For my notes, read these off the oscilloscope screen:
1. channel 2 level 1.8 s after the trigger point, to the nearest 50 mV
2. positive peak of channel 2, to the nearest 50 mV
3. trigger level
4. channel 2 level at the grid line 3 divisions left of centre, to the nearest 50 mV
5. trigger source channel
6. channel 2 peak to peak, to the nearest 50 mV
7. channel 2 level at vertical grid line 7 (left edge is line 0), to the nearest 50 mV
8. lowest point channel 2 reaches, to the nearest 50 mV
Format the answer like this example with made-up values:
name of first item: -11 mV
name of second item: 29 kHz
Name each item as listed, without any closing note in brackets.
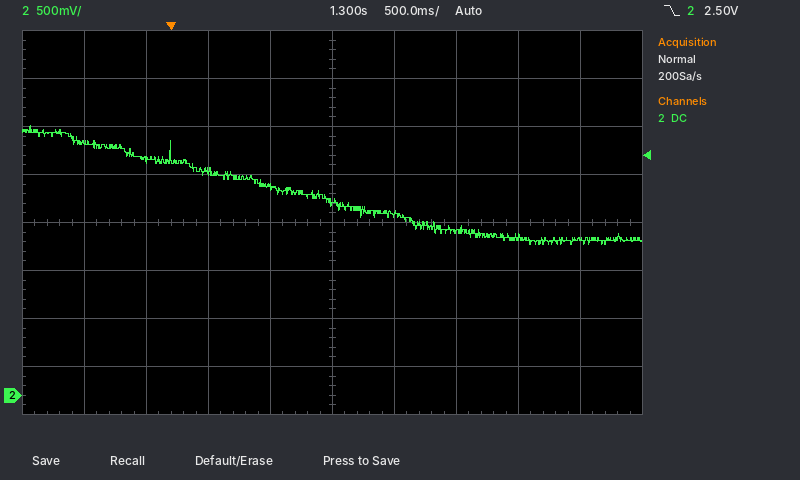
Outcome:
channel 2 level 1.8 s after the trigger point, to the nearest 50 mV: 1.90 V
positive peak of channel 2, to the nearest 50 mV: 2.80 V
trigger level: 2.50 V
channel 2 level at the grid line 3 divisions left of centre, to the nearest 50 mV: 2.45 V
trigger source channel: channel 2
channel 2 peak to peak, to the nearest 50 mV: 1.25 V
channel 2 level at vertical grid line 7 (left edge is line 0), to the nearest 50 mV: 1.70 V
lowest point channel 2 reaches, to the nearest 50 mV: 1.55 V
